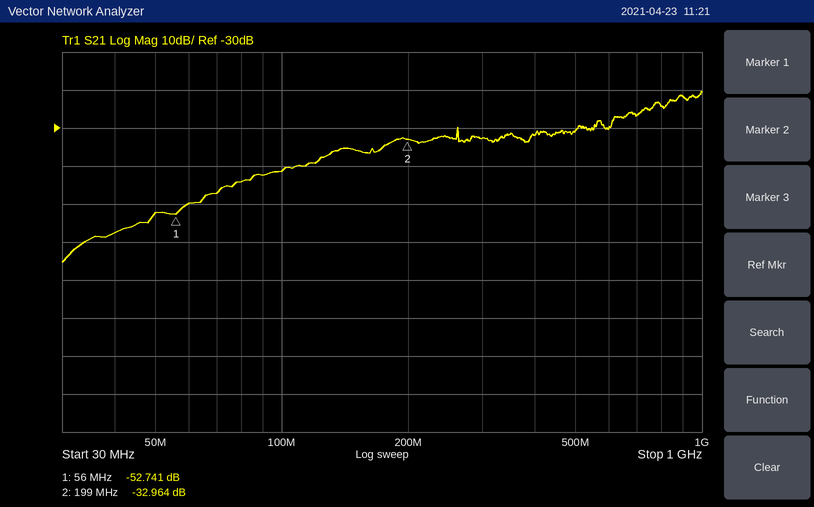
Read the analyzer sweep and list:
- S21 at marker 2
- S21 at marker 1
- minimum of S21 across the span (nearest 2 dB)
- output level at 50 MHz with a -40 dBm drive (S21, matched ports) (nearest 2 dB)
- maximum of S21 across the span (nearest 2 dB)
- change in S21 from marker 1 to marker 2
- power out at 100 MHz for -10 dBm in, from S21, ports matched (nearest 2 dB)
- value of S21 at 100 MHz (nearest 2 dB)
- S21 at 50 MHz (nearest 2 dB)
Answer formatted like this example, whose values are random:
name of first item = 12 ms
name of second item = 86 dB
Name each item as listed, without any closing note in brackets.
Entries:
S21 at marker 2 = -32.964 dB
S21 at marker 1 = -52.741 dB
minimum of S21 across the span = -66 dB
output level at 50 MHz with a -40 dBm drive (S21, matched ports) = -92 dBm
maximum of S21 across the span = -20 dB
change in S21 from marker 1 to marker 2 = 19.777 dB
power out at 100 MHz for -10 dBm in, from S21, ports matched = -52 dBm
value of S21 at 100 MHz = -42 dB
S21 at 50 MHz = -52 dB
